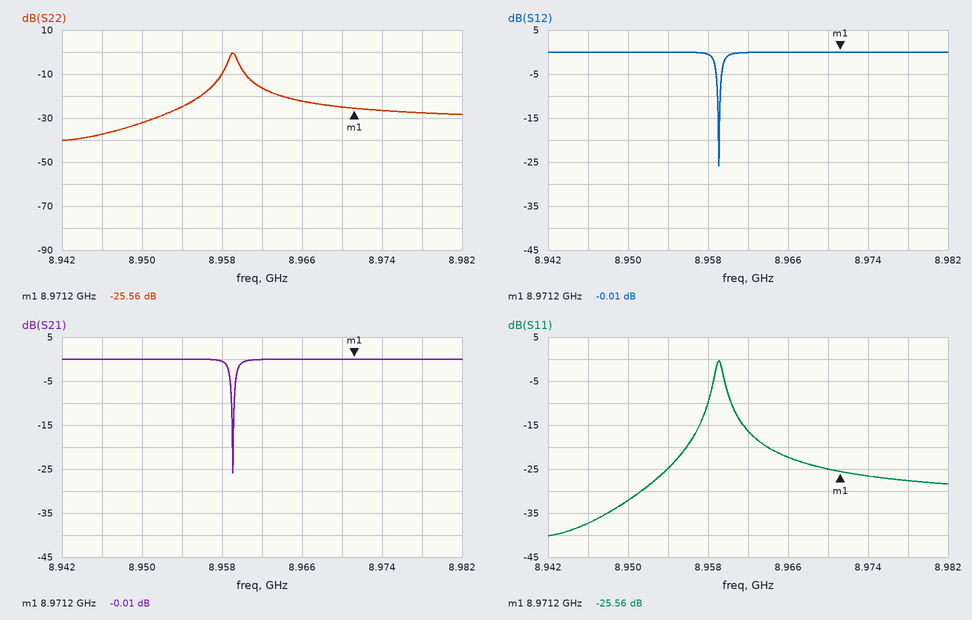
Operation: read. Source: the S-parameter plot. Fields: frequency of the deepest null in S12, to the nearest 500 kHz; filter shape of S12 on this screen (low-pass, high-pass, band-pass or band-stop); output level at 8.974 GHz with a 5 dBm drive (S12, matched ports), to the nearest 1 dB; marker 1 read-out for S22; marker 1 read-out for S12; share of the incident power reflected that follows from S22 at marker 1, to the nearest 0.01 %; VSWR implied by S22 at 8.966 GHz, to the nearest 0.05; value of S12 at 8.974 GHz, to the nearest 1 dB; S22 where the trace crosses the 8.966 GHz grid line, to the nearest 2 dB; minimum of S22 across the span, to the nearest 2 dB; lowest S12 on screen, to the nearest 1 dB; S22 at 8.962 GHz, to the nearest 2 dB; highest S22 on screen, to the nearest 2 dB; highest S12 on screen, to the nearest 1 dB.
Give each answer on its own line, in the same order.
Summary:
8.9590 GHz
band-stop
5 dBm
-25.56 dB
-0.01 dB
0.28 %
1.15
0 dB
-22 dB
-40 dB
-26 dB
-16 dB
0 dB
0 dB
